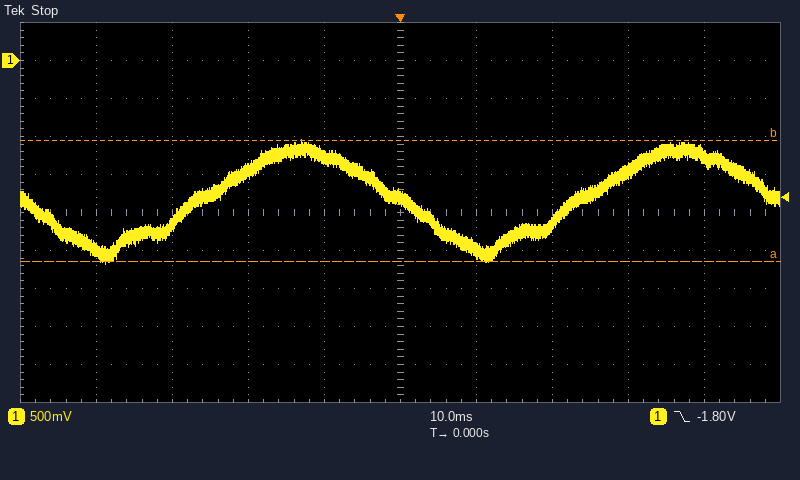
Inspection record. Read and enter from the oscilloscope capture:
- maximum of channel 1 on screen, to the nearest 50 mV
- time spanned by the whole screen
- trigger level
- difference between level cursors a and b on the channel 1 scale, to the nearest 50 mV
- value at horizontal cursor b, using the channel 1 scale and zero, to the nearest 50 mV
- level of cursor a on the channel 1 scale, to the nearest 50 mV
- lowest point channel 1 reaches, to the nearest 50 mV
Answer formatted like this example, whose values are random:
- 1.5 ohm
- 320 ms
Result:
- -1.05 V
- 100 ms
- -1.80 V
- 1.60 V
- -1.05 V
- -2.65 V
- -2.65 V
